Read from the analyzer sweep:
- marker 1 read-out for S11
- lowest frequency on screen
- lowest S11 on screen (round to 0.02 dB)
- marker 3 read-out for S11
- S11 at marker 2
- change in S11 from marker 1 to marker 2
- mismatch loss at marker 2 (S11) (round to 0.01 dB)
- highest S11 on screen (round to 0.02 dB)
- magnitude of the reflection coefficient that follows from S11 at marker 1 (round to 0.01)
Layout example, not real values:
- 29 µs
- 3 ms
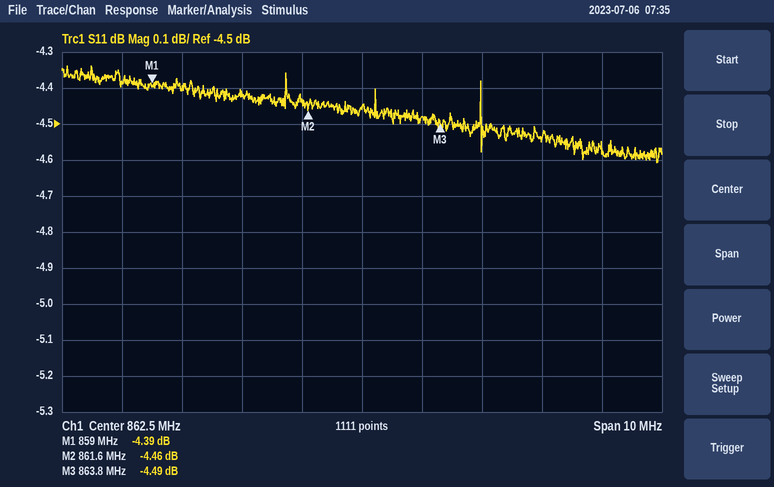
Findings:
- -4.39 dB
- 857.5 MHz
- -4.60 dB
- -4.49 dB
- -4.46 dB
- -0.07 dB
- 1.93 dB
- -4.34 dB
- 0.60
